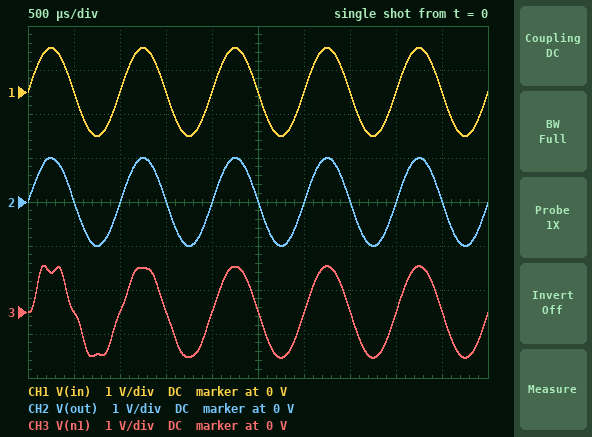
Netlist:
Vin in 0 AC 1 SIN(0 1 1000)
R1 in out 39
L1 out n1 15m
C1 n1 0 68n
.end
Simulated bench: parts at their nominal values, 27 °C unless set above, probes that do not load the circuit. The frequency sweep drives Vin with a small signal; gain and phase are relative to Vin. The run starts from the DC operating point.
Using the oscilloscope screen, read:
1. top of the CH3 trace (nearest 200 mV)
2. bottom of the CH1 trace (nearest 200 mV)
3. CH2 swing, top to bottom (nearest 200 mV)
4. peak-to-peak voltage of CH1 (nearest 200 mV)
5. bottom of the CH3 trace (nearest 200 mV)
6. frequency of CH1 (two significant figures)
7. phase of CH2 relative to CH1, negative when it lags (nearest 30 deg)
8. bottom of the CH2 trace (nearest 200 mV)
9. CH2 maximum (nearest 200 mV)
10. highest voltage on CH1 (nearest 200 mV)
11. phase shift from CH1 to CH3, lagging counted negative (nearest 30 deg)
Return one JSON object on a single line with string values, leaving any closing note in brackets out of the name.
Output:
{"top of the CH3 trace": "1.0 V", "bottom of the CH1 trace": "-1.0 V", "CH2 swing, top to bottom": "2.0 V", "peak-to-peak voltage of CH1": "2.0 V", "bottom of the CH3 trace": "-1.0 V", "frequency of CH1": "1.0 kHz", "phase of CH2 relative to CH1, negative when it lags": "0 deg", "bottom of the CH2 trace": "-1.0 V", "CH2 maximum": "1.0 V", "highest voltage on CH1": "1.0 V", "phase shift from CH1 to CH3, lagging counted negative": "0 deg"}
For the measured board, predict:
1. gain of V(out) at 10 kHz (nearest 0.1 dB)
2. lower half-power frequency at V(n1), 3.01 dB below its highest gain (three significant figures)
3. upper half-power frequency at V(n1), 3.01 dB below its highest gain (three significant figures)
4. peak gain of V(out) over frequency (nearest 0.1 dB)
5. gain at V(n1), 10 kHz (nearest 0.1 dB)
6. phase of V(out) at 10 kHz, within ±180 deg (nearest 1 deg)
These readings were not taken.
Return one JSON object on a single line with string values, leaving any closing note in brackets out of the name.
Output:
{"gain of V(out) at 10 kHz": "0 dB", "lower half-power frequency at V(n1), 3.01 dB below its highest gain": "4.76 kHz", "upper half-power frequency at V(n1), 3.01 dB below its highest gain": "5.18 kHz", "peak gain of V(out) over frequency": "0 dB", "gain at V(n1), 10 kHz": "-9.6 dB", "phase of V(out) at 10 kHz, within ±180 deg": "3 deg"}
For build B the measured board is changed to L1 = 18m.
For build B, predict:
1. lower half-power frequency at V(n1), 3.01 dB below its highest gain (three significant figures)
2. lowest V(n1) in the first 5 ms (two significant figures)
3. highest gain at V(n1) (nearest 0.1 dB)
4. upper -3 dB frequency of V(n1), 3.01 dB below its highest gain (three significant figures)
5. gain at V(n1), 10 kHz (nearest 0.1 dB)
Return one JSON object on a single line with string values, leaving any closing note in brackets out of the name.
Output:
{"lower half-power frequency at V(n1), 3.01 dB below its highest gain": "4.37 kHz", "lowest V(n1) in the first 5 ms": "-1.1 V", "highest gain at V(n1)": "22.4 dB", "upper -3 dB frequency of V(n1), 3.01 dB below its highest gain": "4.71 kHz", "gain at V(n1), 10 kHz": "-11.7 dB"}
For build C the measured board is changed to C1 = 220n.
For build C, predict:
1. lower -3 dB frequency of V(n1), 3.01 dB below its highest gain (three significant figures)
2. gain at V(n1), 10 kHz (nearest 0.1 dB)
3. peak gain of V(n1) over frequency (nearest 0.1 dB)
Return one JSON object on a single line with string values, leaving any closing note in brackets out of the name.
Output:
{"lower -3 dB frequency of V(n1), 3.01 dB below its highest gain": "2.54 kHz", "gain at V(n1), 10 kHz": "-21.6 dB", "peak gain of V(n1) over frequency": "16.5 dB"}
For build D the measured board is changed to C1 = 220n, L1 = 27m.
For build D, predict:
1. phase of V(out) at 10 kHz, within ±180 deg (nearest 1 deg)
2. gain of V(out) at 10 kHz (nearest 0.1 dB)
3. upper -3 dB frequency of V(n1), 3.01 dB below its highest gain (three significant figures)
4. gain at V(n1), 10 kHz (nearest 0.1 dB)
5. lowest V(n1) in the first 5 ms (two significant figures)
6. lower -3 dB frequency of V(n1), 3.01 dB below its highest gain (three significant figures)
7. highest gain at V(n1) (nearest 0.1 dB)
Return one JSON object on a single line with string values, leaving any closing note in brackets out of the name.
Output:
{"phase of V(out) at 10 kHz, within ±180 deg": "1 deg", "gain of V(out) at 10 kHz": "0 dB", "upper -3 dB frequency of V(n1), 3.01 dB below its highest gain": "2.17 kHz", "gain at V(n1), 10 kHz": "-27.0 dB", "lowest V(n1) in the first 5 ms": "-1.4 V", "lower -3 dB frequency of V(n1), 3.01 dB below its highest gain": "1.94 kHz", "highest gain at V(n1)": "19.1 dB"}
